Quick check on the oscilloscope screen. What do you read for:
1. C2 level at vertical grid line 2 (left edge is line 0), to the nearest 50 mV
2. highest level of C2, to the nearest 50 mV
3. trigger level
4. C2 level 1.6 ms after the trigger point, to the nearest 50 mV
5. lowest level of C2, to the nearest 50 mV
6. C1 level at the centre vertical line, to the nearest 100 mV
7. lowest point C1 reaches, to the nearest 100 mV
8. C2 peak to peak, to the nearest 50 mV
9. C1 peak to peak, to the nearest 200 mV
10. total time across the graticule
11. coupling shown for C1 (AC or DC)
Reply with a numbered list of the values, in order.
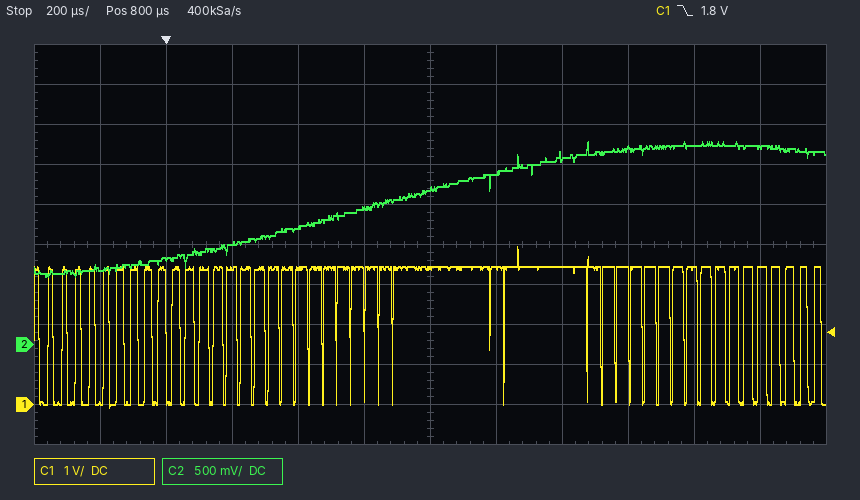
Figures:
1. 1.05 V
2. 2.55 V
3. 1.8 V
4. 2.50 V
5. 850 mV
6. 3.4 V
7. -100 mV
8. 1.70 V
9. 4.0 V
10. 2.4 ms
11. DC
